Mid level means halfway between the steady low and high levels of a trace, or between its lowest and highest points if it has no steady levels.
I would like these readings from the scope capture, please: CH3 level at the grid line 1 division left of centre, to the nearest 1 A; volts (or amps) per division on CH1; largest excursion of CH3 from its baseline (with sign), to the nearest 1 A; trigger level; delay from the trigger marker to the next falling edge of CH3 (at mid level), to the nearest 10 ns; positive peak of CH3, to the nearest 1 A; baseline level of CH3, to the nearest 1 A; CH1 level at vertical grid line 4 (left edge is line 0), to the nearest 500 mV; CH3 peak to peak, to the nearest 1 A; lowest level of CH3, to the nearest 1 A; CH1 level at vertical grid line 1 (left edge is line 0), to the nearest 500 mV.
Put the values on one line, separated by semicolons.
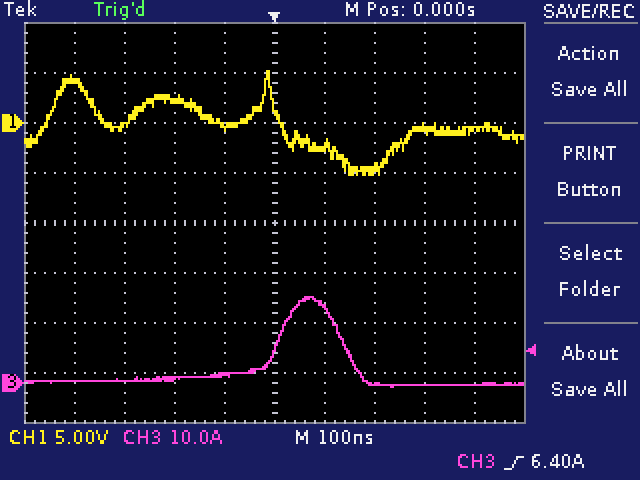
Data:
2 A; 5 V; +17 A; 6.40 A; 140 ns; 17 A; 0 A; -500 mV; 18 A; -1 A; 4.5 V
